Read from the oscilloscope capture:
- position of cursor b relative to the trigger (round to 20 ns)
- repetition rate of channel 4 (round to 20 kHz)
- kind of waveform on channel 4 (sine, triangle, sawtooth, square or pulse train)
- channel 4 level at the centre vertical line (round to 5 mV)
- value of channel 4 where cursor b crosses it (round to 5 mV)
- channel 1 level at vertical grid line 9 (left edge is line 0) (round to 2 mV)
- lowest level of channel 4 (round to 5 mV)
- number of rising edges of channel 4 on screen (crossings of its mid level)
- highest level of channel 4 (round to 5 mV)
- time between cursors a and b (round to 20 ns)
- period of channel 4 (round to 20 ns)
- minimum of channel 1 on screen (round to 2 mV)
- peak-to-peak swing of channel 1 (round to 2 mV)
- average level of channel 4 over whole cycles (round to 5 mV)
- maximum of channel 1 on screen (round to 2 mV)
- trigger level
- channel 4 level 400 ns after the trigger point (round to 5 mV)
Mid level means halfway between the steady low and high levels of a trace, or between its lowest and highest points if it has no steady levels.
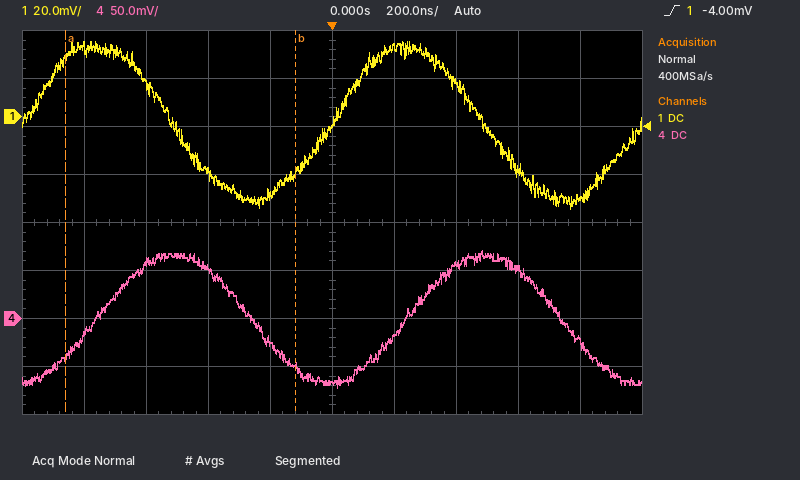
-120 ns
1.00 MHz
sine
-65 mV
-50 mV
-34 mV
-70 mV
2
70 mV
740 ns
1.00 µs
-38 mV
70 mV
0 mV
32 mV
-4.00 mV
55 mV
